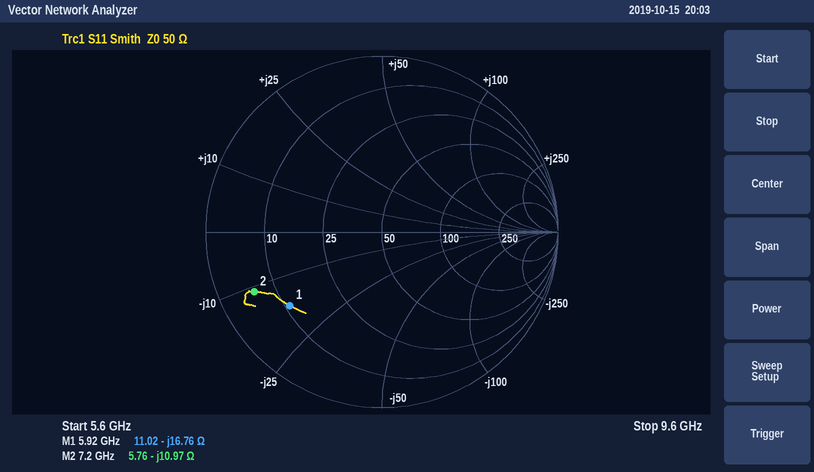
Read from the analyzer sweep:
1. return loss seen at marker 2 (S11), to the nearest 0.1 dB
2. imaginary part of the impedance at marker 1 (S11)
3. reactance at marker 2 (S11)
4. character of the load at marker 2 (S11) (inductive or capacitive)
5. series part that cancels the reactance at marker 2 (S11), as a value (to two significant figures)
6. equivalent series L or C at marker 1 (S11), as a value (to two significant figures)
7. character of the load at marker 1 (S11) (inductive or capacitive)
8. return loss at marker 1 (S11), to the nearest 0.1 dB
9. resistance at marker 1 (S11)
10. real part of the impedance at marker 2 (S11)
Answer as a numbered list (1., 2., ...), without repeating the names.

1. 1.9 dB
2. -16.76 Ω
3. -10.97 Ω
4. capacitive
5. 240 pH
6. 1.6 pF
7. capacitive
8. 3.5 dB
9. 11.02 Ω
10. 5.76 Ω
